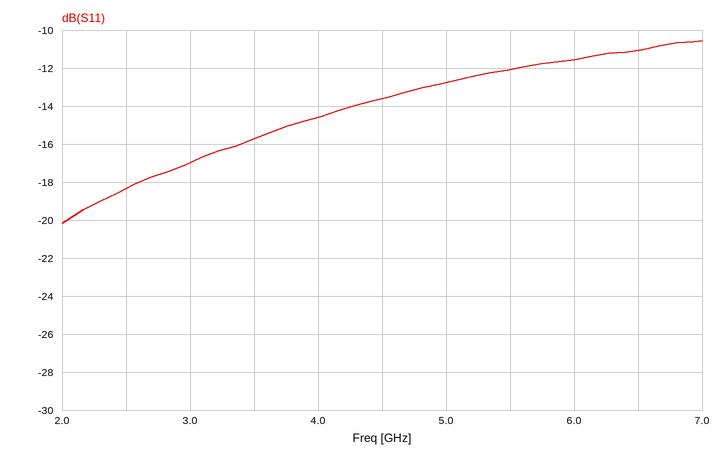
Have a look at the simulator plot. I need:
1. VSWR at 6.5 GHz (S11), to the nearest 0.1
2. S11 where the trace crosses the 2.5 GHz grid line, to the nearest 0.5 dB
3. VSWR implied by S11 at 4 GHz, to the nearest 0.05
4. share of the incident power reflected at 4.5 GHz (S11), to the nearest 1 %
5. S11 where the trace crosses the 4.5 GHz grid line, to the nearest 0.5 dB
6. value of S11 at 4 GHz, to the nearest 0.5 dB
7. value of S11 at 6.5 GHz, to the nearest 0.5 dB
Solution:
1.8
-18.5 dB
1.45
4 %
-13.5 dB
-14.5 dB
-11.0 dB
